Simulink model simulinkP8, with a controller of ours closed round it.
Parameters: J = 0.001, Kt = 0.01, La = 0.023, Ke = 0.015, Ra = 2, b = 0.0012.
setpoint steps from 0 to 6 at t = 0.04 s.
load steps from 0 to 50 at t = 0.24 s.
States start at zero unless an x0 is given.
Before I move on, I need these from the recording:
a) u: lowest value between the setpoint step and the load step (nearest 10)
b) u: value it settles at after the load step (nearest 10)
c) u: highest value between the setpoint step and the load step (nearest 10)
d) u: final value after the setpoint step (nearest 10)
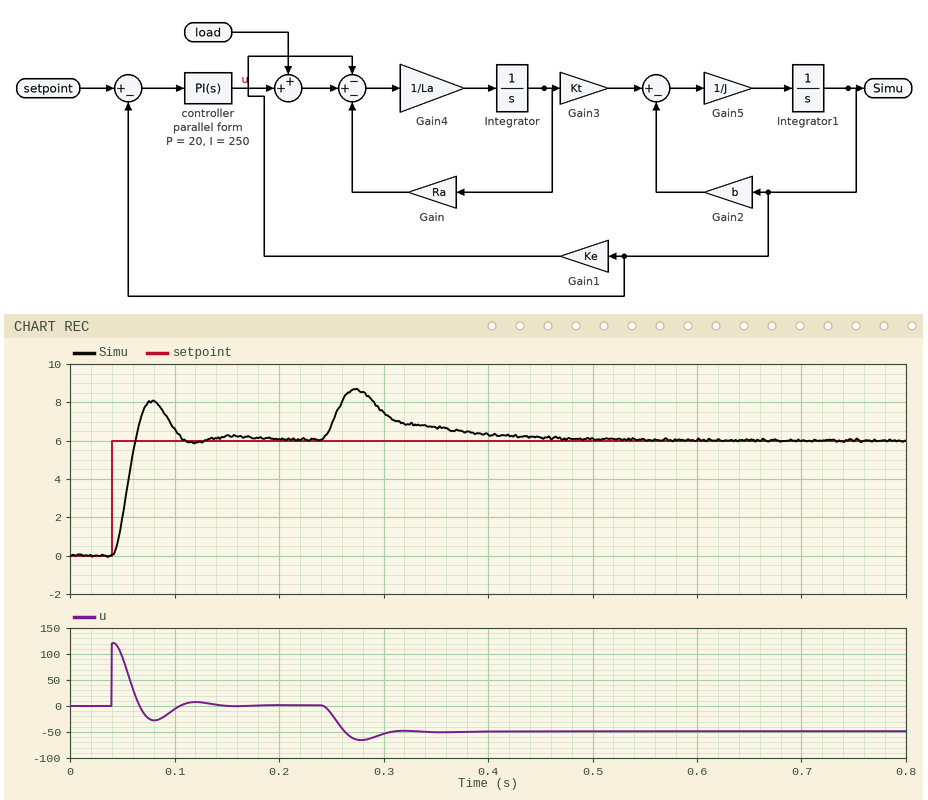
-30
-50
120
0
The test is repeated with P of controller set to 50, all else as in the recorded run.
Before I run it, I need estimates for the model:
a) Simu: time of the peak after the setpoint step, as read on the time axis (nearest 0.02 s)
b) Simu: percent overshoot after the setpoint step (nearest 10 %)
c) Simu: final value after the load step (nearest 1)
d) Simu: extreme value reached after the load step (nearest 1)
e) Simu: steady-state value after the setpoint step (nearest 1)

0.06 s
40 %
6
7
6
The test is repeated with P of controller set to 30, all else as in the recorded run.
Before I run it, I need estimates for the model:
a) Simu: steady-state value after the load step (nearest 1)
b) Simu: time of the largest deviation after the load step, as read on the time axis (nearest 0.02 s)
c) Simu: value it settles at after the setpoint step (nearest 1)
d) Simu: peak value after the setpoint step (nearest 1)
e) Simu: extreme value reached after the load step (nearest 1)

6
0.26 s
6
8
8
